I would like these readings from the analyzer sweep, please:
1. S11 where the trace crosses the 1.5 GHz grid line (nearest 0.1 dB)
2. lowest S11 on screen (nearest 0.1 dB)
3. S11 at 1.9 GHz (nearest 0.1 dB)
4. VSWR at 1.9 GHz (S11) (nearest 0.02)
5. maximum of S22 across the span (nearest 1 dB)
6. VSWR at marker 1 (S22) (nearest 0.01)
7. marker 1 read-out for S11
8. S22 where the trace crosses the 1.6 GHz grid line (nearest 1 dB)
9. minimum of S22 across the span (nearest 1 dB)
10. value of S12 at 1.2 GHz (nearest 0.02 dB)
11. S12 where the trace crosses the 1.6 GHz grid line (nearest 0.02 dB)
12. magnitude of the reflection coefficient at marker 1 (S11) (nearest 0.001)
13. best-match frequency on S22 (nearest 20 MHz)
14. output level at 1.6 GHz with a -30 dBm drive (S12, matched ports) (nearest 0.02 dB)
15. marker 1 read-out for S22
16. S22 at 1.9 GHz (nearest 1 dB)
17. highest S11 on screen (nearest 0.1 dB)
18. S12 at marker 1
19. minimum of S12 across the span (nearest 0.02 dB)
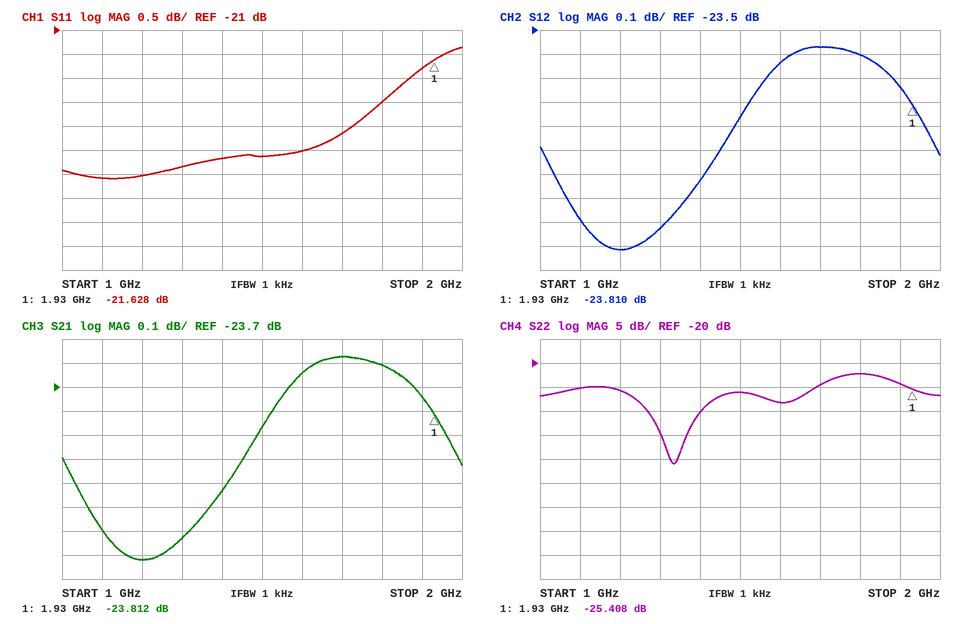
-23.6 dB
-24.1 dB
-21.8 dB
1.18
-22 dB
1.11
-21.628 dB
-28 dB
-41 dB
-24.42 dB
-23.64 dB
0.083
1.34 GHz
-53.64 dBm
-25.408 dB
-24 dB
-21.4 dB
-23.810 dB
-24.42 dB
